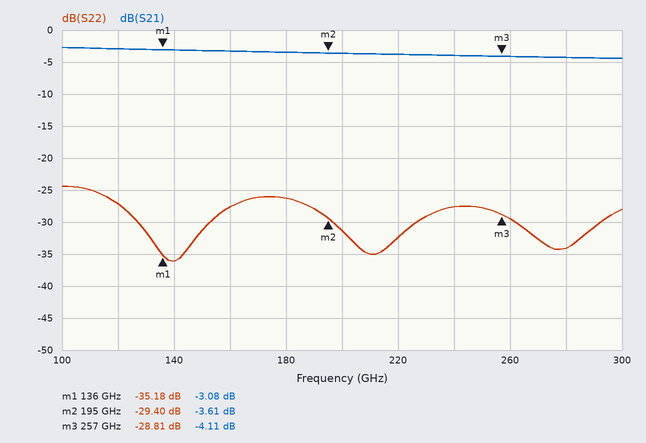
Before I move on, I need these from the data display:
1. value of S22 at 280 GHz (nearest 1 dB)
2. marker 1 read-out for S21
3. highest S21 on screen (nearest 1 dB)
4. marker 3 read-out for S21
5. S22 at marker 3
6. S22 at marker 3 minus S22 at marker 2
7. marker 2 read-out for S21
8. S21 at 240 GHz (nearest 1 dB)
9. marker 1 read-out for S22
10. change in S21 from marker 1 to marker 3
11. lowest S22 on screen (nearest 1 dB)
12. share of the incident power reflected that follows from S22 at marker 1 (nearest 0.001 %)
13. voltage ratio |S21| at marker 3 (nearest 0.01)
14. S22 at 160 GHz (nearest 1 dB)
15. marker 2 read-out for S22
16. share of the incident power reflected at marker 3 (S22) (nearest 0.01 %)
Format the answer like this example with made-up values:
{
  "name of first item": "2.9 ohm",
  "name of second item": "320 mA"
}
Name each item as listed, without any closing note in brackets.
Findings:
{
  "value of S22 at 280 GHz": "-34 dB",
  "marker 1 read-out for S21": "-3.08 dB",
  "highest S21 on screen": "-3 dB",
  "marker 3 read-out for S21": "-4.11 dB",
  "S22 at marker 3": "-28.81 dB",
  "S22 at marker 3 minus S22 at marker 2": "0.59 dB",
  "marker 2 read-out for S21": "-3.61 dB",
  "S21 at 240 GHz": "-4 dB",
  "marker 1 read-out for S22": "-35.18 dB",
  "change in S21 from marker 1 to marker 3": "-1.03 dB",
  "lowest S22 on screen": "-36 dB",
  "share of the incident power reflected that follows from S22 at marker 1": "0.030 %",
  "voltage ratio |S21| at marker 3": "0.62",
  "S22 at 160 GHz": "-28 dB",
  "marker 2 read-out for S22": "-29.40 dB",
  "share of the incident power reflected at marker 3 (S22)": "0.13 %"
}
